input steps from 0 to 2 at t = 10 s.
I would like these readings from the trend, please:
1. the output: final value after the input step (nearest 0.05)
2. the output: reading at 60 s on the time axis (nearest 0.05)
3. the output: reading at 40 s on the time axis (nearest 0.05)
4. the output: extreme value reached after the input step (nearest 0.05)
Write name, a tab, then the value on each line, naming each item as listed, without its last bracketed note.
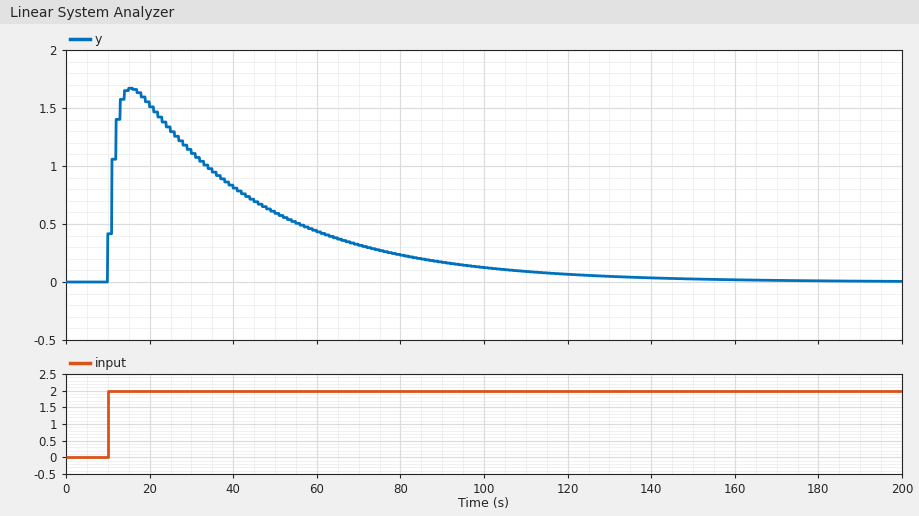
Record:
the output: final value after the input step	0.00
the output: reading at 60 s on the time axis	0.45
the output: reading at 40 s on the time axis	0.80
the output: extreme value reached after the input step	1.65
